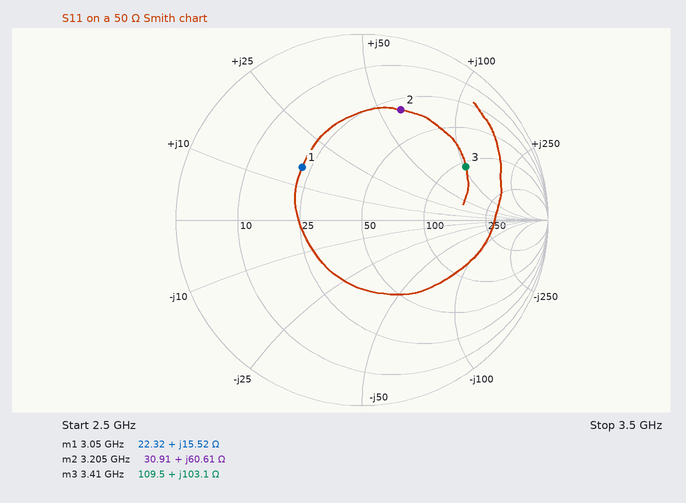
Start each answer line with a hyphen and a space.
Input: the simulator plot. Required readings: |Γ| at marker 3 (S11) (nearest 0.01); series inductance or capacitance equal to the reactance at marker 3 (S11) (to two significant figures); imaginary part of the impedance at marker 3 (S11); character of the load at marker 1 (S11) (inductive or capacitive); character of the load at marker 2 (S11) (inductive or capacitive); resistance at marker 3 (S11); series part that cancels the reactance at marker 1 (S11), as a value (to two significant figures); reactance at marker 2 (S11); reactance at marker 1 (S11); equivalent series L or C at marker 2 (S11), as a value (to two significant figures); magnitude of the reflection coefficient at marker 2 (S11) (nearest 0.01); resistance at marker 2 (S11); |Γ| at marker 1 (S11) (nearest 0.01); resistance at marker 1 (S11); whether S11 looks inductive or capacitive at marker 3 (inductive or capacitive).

- 0.63
- 4.8 nH
- +103.1 Ω
- inductive
- inductive
- 109.5 Ω
- 3.4 pF
- +60.61 Ω
- +15.52 Ω
- 3.0 nH
- 0.63
- 30.91 Ω
- 0.43
- 22.32 Ω
- inductive
